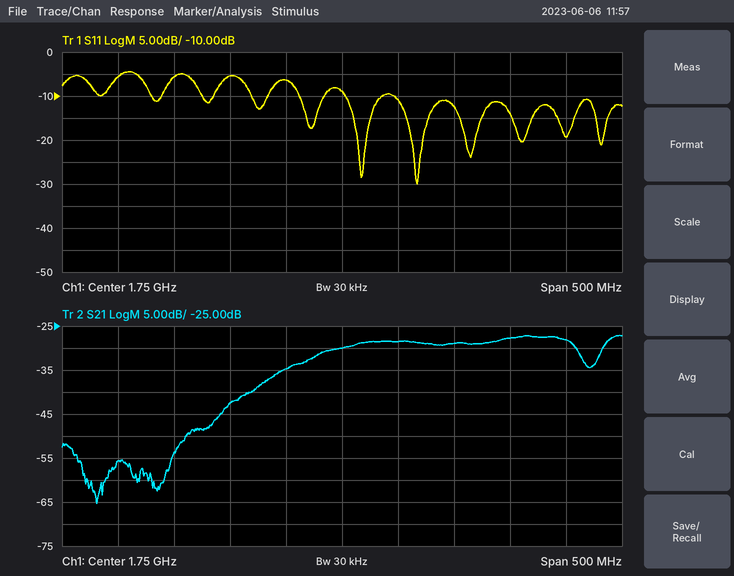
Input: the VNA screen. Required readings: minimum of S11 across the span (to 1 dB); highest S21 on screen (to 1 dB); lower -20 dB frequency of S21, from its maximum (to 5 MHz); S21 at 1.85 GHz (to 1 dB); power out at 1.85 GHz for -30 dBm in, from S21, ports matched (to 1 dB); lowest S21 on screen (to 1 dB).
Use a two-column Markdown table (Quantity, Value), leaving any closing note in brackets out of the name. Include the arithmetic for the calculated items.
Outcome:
| Quantity | Value |
|---|---|
| minimum of S11 across the span | -30 dB |
| highest S21 on screen | -27 dB |
| lower -20 dB frequency of S21, from its maximum | 1.635 GHz |
| S21 at 1.85 GHz | -29 dB |
| power out at 1.85 GHz for -30 dBm in, from S21, ports matched | -30 dBm + (-29 dB) = -59 dBm |
| lowest S21 on screen | -65 dB |
